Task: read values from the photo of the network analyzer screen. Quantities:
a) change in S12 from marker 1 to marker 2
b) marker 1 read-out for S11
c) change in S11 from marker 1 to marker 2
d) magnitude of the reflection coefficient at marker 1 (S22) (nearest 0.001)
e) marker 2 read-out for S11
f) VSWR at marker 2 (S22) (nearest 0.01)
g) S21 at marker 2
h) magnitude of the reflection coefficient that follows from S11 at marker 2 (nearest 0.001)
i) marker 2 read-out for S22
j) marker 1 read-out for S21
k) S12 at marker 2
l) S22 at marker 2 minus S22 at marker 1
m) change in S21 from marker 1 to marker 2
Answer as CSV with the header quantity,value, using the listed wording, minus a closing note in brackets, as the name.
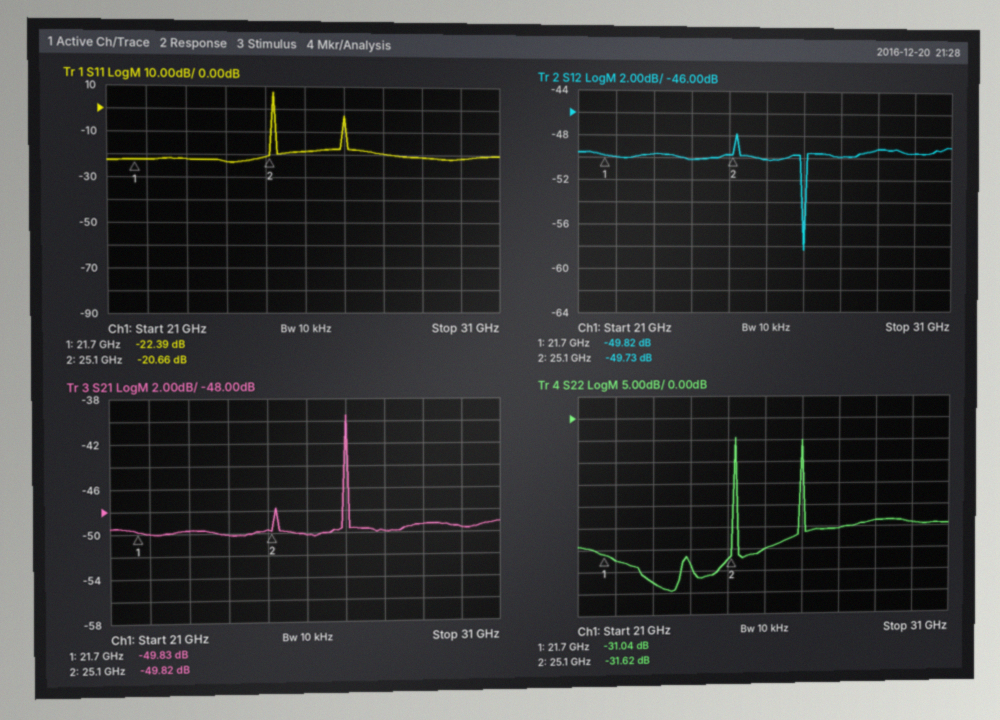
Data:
quantity,value
change in S12 from marker 1 to marker 2,0.09 dB
marker 1 read-out for S11,-22.39 dB
change in S11 from marker 1 to marker 2,1.73 dB
magnitude of the reflection coefficient at marker 1 (S22),0.028
marker 2 read-out for S11,-20.66 dB
VSWR at marker 2 (S22),1.05
S21 at marker 2,-49.82 dB
magnitude of the reflection coefficient that follows from S11 at marker 2,0.093
marker 2 read-out for S22,-31.62 dB
marker 1 read-out for S21,-49.83 dB
S12 at marker 2,-49.73 dB
S22 at marker 2 minus S22 at marker 1,-0.58 dB
change in S21 from marker 1 to marker 2,0.01 dB
